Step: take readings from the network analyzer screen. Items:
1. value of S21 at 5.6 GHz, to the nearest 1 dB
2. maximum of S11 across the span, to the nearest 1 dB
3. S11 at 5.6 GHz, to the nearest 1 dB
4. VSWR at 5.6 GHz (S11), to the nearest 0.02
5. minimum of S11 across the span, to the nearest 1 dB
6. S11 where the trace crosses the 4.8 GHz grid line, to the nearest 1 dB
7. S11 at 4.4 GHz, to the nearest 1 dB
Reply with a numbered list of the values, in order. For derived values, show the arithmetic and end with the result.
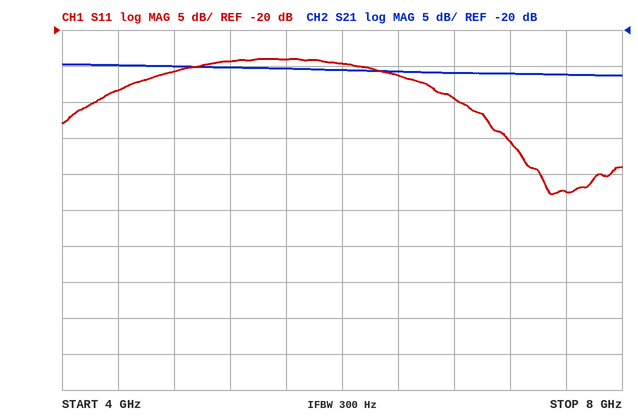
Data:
1. -25 dB
2. -24 dB
3. -24 dB
4. |Γ| = 10^(-24/20) = 0.0631; VSWR = (1 + 0.0631)/(1 − 0.0631) ≈ 1.13, so 1.14 to the nearest 0.02
5. -43 dB
6. -26 dB
7. -28 dB
